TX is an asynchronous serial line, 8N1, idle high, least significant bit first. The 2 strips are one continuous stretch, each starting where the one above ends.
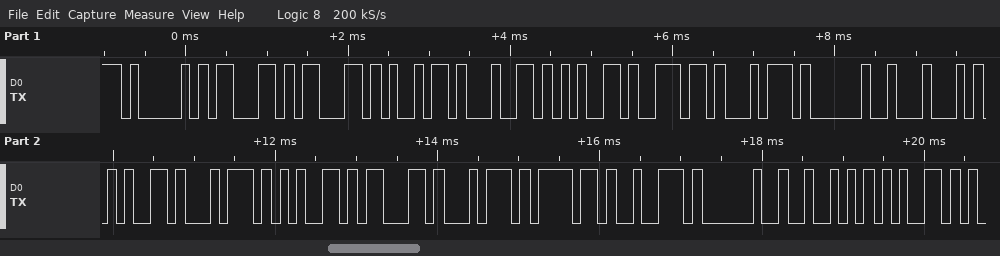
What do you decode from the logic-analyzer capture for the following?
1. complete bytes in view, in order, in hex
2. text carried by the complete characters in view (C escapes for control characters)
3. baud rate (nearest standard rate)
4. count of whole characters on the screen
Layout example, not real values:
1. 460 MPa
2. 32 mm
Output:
1. 41 63 63 69 64 65 6E 74 20 44 65 74 65 63 74 6F 72 20 52 65
2. "Accident Detector Re"
3. 9600 baud
4. 20
